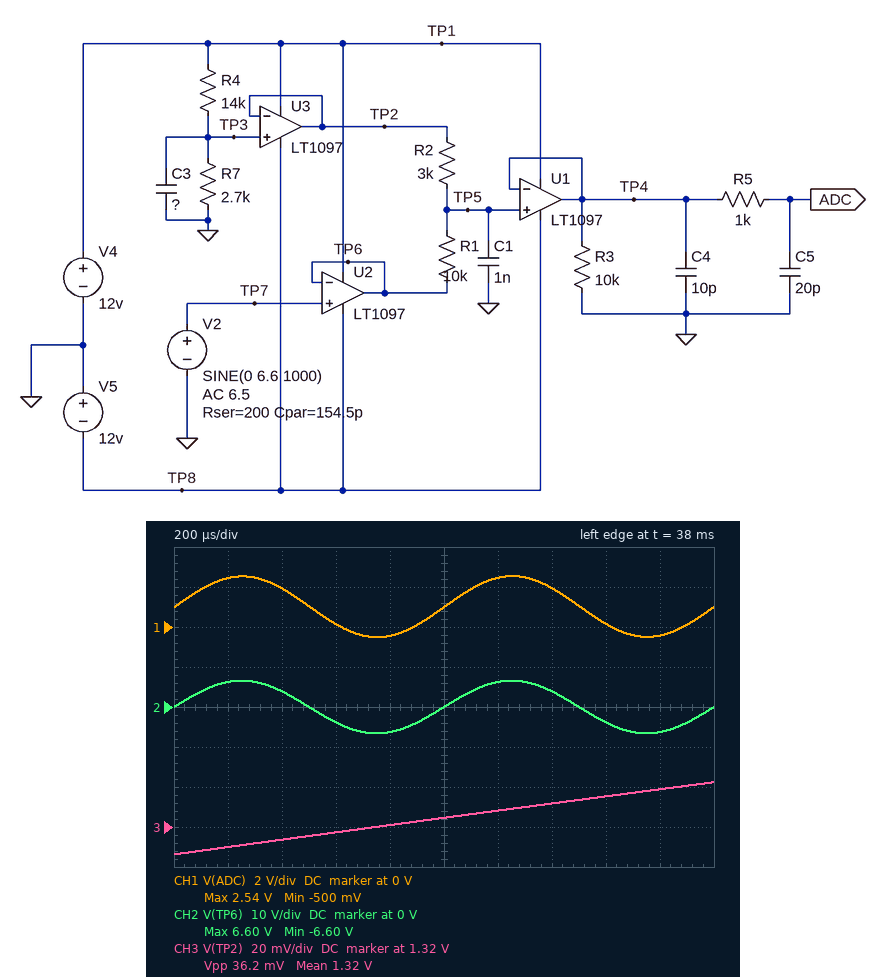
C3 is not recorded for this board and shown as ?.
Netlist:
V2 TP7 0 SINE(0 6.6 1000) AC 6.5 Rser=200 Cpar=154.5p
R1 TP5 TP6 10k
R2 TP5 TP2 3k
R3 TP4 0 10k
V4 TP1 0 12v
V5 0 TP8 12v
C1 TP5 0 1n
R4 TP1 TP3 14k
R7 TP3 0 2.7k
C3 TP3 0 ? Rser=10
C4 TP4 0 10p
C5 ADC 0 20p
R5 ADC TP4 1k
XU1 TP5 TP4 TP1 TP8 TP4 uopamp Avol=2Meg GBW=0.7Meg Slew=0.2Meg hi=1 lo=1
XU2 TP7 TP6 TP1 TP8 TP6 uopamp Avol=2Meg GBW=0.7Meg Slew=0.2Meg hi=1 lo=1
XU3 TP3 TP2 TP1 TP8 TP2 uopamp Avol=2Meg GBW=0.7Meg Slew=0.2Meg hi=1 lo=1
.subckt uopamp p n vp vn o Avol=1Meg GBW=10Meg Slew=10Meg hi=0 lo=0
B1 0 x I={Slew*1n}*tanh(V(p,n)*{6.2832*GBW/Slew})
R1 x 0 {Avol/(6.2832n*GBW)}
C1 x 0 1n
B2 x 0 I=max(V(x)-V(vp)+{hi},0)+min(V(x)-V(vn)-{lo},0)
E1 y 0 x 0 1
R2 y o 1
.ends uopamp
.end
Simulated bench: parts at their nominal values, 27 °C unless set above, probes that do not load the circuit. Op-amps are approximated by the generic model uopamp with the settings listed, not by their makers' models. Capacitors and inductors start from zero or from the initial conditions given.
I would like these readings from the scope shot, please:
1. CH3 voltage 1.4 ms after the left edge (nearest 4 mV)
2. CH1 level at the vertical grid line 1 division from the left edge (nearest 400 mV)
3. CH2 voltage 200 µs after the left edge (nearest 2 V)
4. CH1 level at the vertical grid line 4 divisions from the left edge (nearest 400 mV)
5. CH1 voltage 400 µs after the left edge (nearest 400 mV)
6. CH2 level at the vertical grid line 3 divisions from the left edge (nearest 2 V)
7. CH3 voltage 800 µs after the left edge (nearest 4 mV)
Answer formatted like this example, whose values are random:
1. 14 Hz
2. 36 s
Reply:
1. 1.332 V
2. 2.4 V
3. 6 V
4. -400 mV
5. 2.0 V
6. -4 V
7. 1.320 V
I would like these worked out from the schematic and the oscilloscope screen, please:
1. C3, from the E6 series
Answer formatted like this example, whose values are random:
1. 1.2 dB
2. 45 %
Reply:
1. 15 µF
